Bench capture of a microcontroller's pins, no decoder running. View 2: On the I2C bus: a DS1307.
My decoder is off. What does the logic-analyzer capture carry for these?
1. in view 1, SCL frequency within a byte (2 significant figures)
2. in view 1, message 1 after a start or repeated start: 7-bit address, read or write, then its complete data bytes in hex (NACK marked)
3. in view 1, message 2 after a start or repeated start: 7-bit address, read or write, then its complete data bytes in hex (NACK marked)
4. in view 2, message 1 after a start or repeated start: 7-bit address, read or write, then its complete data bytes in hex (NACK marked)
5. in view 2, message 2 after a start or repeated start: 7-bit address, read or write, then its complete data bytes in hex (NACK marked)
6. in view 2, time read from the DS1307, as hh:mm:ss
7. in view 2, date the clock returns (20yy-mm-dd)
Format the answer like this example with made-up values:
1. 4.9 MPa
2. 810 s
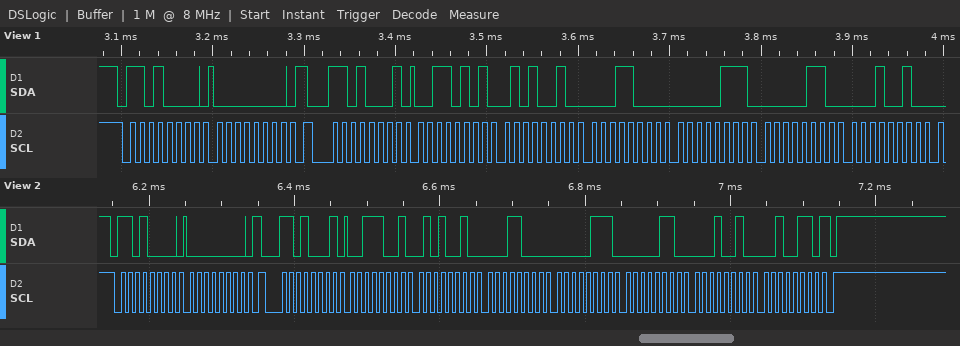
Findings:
1. 100 kHz
2. 0x68 write: 00
3. 0x68 read: 35 52 18 07 06 12
4. 0x68 write: 00
5. 0x68 read: 39 52 18 07 06 12 26 NACK
6. 18:52:39
7. 2026-12-06
